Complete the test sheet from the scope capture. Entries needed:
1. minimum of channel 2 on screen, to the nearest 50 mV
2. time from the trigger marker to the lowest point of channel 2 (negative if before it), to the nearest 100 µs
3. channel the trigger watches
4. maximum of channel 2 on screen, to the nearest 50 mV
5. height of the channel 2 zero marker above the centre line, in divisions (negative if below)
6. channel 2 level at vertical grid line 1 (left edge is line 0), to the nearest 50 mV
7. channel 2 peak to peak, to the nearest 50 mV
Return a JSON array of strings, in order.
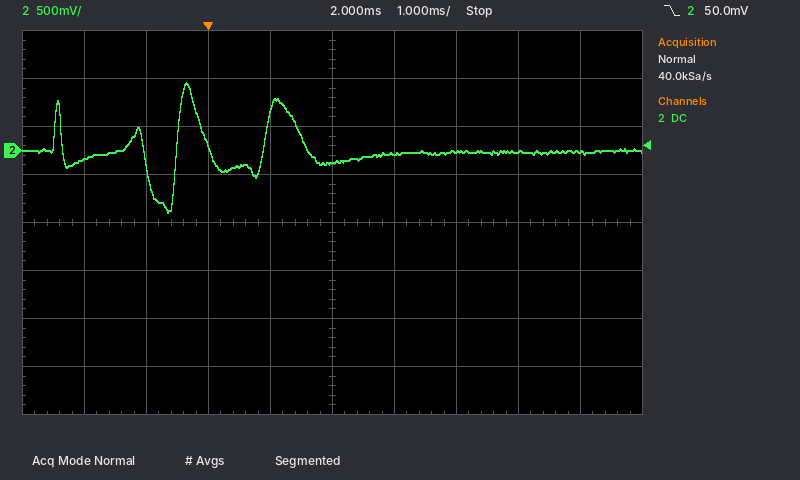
["-650 mV", "-600 µs", "channel 2", "700 mV", "+1.5 div", "-100 mV", "1.35 V"]
